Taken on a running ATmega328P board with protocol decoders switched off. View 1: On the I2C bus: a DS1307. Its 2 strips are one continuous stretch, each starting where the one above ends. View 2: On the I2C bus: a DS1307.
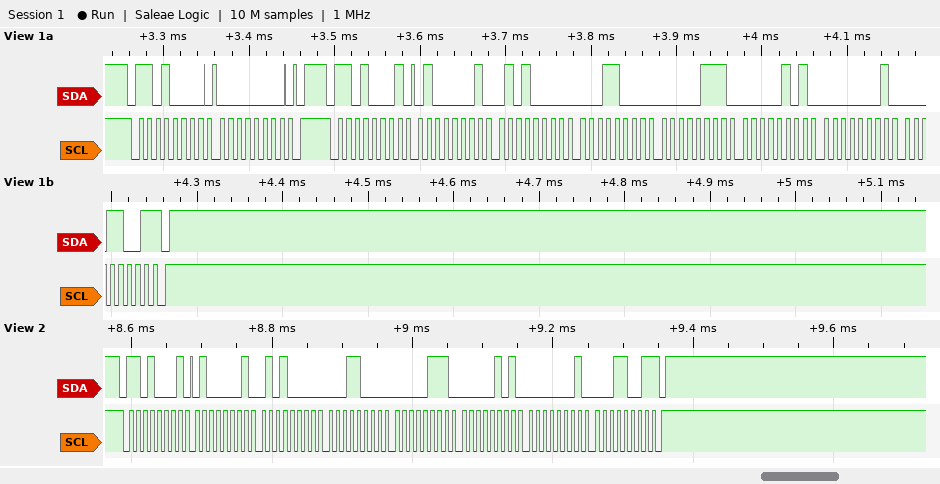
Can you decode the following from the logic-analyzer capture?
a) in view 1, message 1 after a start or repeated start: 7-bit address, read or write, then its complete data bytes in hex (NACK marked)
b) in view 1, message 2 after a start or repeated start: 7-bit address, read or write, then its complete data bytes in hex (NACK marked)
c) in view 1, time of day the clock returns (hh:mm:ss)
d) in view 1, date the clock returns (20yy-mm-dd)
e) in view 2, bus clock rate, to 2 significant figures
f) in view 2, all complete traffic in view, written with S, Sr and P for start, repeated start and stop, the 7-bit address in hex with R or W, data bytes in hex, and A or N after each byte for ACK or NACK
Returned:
0x68 write: 00
0x68 read: 41 50 18 07 05 01 19 NACK
18:50:41
2019-01-05
100 kHz
S 68R A 41 A 50 A 18 A 07 A 05 A 01 A 19 N P
